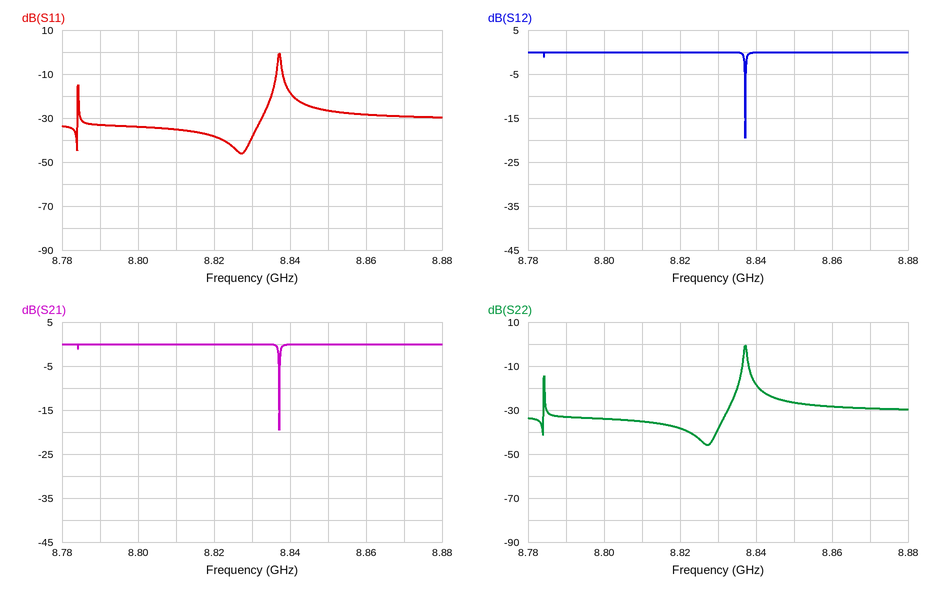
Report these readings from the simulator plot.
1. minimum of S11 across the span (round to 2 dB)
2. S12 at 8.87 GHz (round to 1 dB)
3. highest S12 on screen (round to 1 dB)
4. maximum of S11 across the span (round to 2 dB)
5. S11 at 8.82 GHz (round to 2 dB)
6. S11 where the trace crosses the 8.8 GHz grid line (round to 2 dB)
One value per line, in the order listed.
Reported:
-46 dB
0 dB
0 dB
0 dB
-38 dB
-34 dB
